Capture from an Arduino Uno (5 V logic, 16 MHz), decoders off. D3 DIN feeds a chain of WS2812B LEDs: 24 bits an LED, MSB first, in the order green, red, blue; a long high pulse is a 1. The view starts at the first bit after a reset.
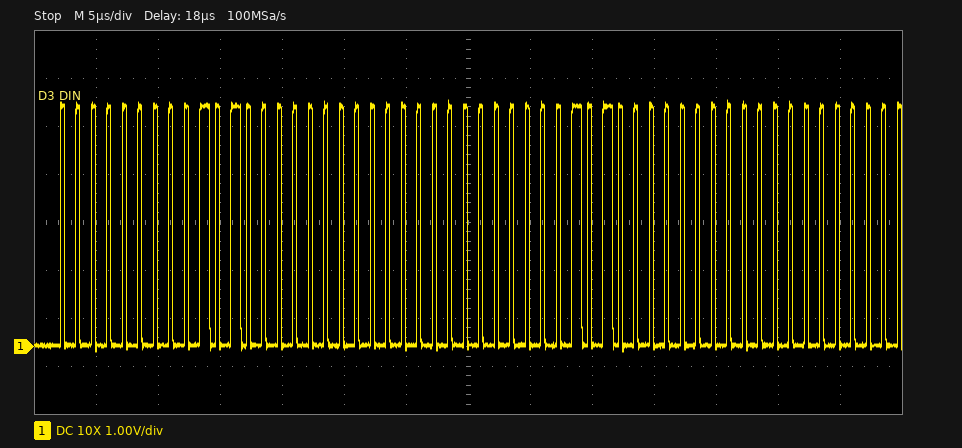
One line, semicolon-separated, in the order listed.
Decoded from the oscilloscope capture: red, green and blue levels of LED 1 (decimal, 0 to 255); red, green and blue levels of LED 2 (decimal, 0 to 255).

80, 0, 0; 80, 0, 0
